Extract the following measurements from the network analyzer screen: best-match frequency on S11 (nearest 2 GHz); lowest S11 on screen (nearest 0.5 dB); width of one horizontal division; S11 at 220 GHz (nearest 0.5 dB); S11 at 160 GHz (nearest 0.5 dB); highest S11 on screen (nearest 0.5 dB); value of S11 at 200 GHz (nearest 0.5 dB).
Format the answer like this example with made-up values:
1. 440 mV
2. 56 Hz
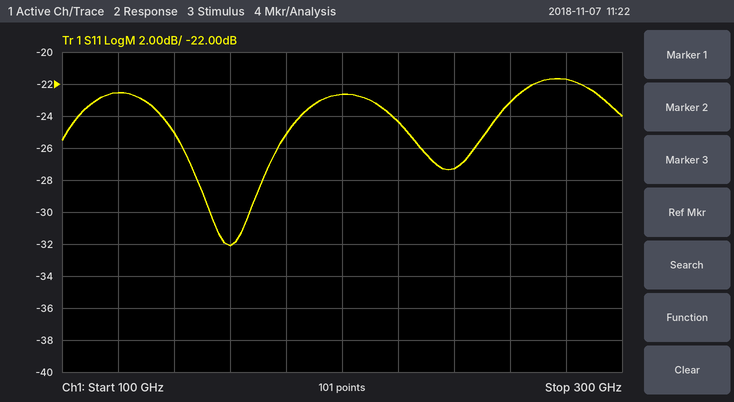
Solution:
1. 160 GHz
2. -32.0 dB
3. 20 GHz
4. -24.5 dB
5. -32.0 dB
6. -21.5 dB
7. -22.5 dB
